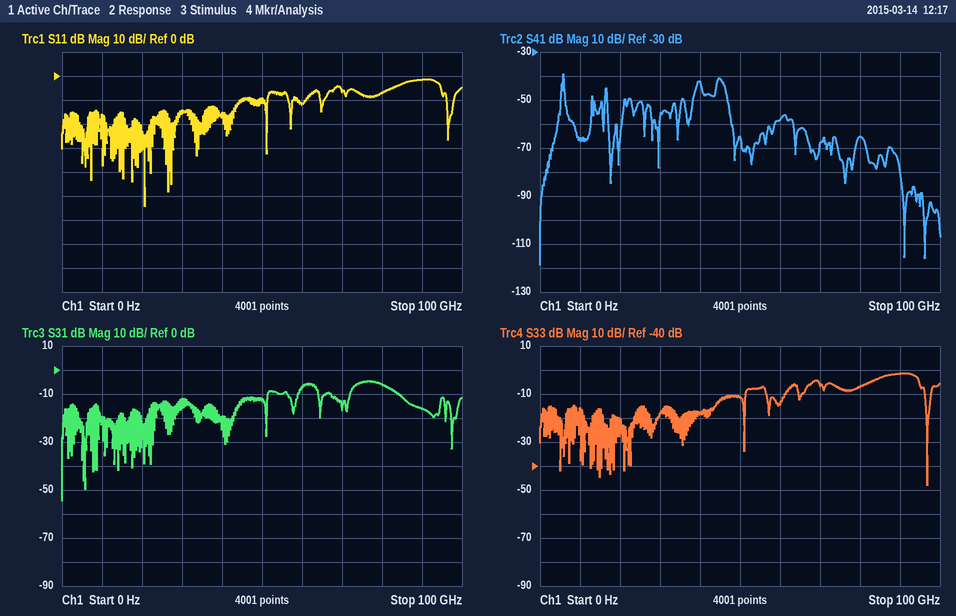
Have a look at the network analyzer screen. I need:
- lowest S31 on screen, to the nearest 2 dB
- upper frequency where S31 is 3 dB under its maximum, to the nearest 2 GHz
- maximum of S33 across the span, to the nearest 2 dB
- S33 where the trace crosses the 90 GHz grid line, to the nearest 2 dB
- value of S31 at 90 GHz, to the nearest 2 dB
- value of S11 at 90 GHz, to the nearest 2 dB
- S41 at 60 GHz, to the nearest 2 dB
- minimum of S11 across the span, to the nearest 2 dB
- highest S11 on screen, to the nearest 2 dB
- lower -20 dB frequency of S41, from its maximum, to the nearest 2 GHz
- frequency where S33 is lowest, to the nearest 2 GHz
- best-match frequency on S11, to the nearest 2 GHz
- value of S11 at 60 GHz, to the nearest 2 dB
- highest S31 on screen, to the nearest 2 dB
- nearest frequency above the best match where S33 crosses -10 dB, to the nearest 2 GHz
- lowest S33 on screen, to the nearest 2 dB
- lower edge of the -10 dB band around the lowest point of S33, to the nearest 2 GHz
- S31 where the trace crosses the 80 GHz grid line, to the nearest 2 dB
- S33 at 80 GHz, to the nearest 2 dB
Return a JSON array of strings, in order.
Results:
["-54 dB", "82 GHz", "-2 dB", "-2 dB", "-16 dB", "-2 dB", "-58 dB", "-54 dB", "-2 dB", "4 GHz", "96 GHz", "20 GHz", "-12 dB", "-4 dB", "98 GHz", "-48 dB", "96 GHz", "-6 dB", "-6 dB"]
